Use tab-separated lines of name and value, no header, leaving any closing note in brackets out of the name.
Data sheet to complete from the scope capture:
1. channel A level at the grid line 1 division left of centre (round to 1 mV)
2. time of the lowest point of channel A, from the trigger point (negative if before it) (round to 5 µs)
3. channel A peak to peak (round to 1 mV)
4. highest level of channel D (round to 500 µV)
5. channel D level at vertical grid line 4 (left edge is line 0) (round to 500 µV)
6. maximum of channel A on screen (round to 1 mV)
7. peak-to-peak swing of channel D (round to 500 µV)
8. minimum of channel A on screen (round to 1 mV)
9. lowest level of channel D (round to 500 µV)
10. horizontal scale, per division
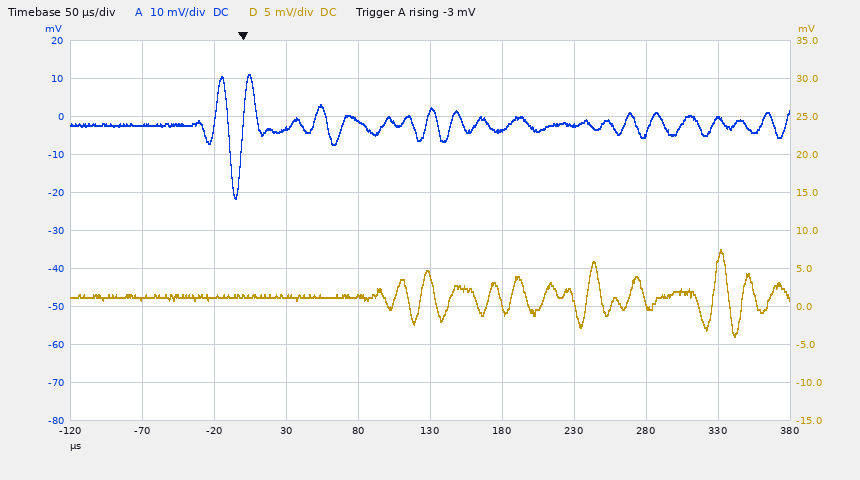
channel A level at the grid line 1 division left of centre	-1 mV
time of the lowest point of channel A, from the trigger point (negative if before it)	-5 µs
channel A peak to peak	33 mV
highest level of channel D	7.5 mV
channel D level at vertical grid line 4 (left edge is line 0)	1.5 mV
maximum of channel A on screen	11 mV
peak-to-peak swing of channel D	11.5 mV
minimum of channel A on screen	-22 mV
lowest level of channel D	-4.0 mV
horizontal scale, per division	50 µs
